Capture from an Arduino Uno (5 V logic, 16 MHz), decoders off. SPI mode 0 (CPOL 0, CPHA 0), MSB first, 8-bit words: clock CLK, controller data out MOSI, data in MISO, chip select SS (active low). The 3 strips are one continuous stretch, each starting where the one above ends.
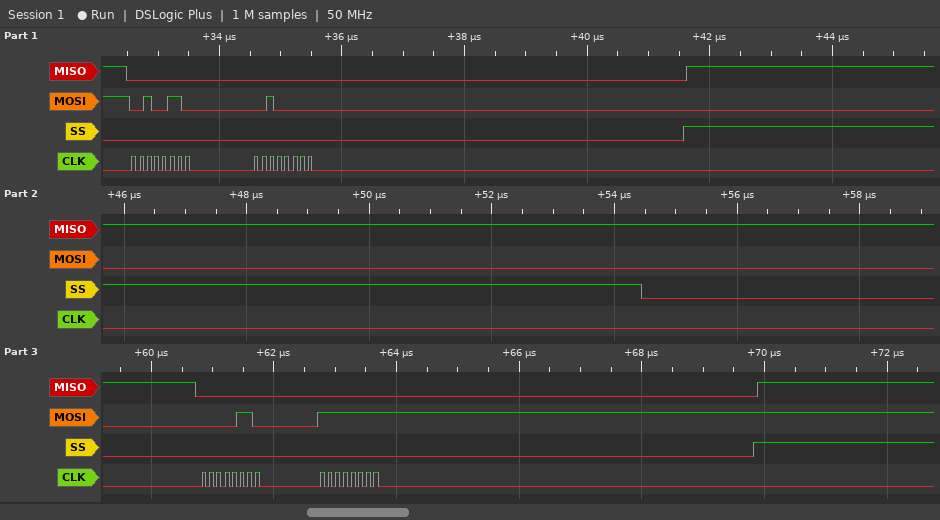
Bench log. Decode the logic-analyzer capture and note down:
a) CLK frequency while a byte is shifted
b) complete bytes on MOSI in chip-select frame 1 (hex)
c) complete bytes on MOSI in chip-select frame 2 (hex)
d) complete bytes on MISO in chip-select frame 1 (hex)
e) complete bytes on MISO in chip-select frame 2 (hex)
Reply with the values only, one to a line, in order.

8 MHz
0x26 0x20
0x06 0xFF
0x00 0x00
0x00 0x00
